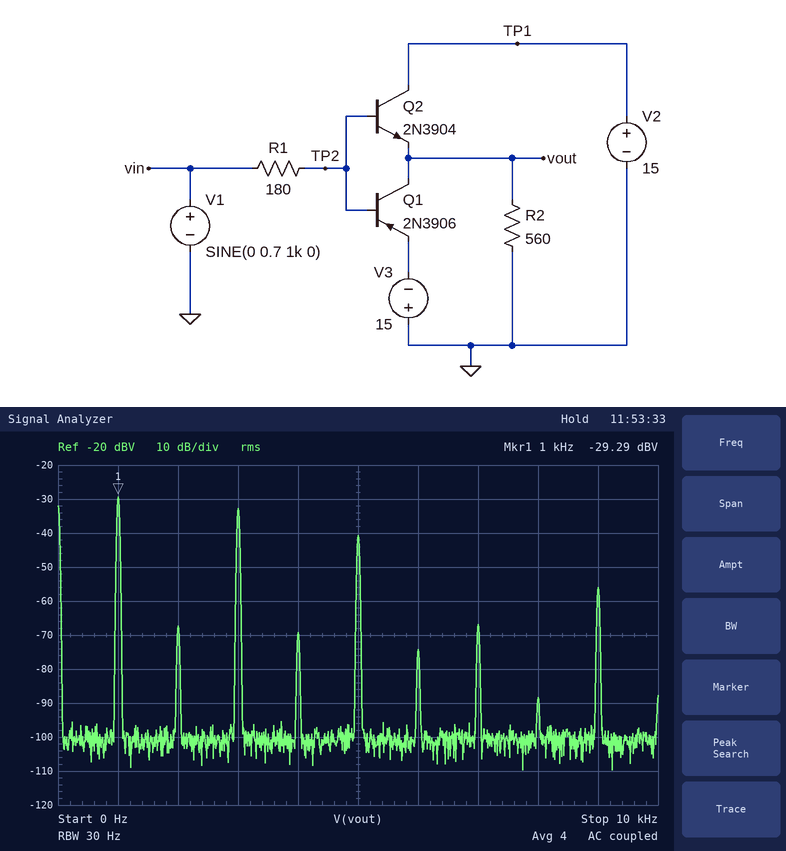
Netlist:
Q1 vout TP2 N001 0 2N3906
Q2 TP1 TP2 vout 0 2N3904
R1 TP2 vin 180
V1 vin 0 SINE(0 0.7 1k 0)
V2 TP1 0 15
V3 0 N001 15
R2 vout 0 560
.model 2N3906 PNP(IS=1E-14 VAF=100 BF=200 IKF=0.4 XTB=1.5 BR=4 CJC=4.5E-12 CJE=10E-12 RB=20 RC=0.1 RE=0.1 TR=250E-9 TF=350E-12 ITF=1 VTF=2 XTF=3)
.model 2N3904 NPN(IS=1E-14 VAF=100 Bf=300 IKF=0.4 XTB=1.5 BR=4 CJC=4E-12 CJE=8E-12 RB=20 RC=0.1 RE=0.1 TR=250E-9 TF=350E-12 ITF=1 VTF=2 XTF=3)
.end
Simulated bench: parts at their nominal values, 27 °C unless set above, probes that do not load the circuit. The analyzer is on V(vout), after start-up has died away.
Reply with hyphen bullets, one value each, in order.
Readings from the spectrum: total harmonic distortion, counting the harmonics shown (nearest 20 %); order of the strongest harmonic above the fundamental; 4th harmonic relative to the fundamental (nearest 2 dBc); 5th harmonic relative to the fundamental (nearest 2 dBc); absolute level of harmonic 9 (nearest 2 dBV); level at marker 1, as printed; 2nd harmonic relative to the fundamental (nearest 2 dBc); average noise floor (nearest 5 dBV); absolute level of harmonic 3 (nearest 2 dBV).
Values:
- 80 %
- 3
- -40 dBc
- -12 dBc
- -56 dBV
- -29.29 dBV
- -38 dBc
- -100 dBV
- -32 dBV
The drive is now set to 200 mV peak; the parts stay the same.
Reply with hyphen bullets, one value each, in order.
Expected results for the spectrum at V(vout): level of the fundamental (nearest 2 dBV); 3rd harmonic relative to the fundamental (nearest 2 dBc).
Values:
- -104 dBV
- -48 dBc
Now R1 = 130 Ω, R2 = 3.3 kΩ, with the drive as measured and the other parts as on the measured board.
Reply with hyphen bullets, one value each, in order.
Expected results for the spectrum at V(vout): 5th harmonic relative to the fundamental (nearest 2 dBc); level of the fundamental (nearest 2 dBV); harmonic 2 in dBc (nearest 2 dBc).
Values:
- -16 dBc
- -26 dBV
- -48 dBc
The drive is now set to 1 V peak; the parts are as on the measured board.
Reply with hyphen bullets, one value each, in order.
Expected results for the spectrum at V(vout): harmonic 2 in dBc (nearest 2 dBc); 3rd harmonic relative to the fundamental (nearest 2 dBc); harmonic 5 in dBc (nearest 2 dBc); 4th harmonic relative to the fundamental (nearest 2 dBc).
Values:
- -34 dBc
- -8 dBc
- -38 dBc
- -44 dBc
